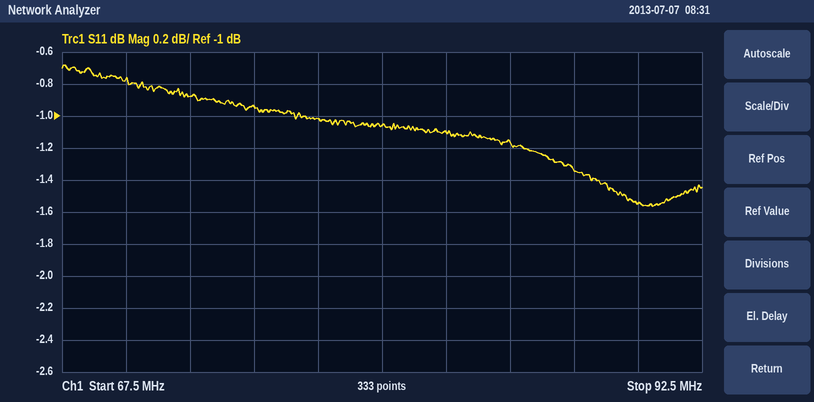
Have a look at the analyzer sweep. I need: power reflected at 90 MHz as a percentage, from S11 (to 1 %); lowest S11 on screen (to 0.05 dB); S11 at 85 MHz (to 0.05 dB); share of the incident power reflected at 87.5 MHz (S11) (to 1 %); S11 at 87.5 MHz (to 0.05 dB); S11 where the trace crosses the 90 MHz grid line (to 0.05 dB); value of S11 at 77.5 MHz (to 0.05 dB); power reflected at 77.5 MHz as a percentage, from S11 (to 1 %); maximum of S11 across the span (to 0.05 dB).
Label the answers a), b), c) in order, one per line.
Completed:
a) 70 %
b) -1.55 dB
c) -1.15 dB
d) 73 %
e) -1.35 dB
f) -1.55 dB
g) -1.00 dB
h) 79 %
i) -0.70 dB
